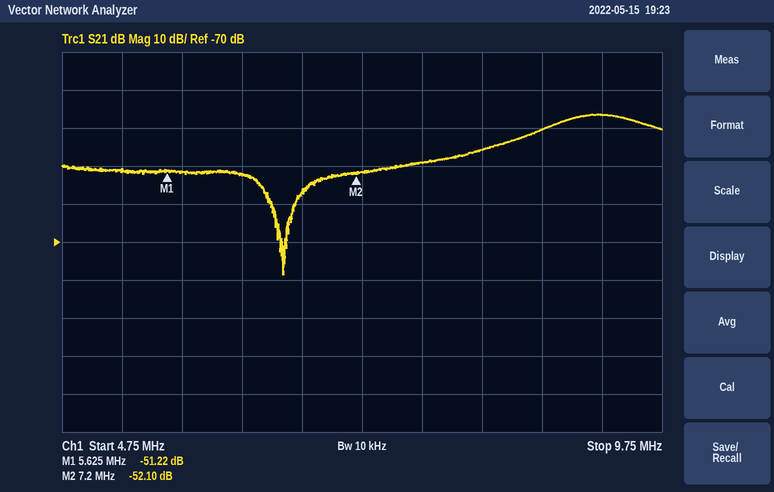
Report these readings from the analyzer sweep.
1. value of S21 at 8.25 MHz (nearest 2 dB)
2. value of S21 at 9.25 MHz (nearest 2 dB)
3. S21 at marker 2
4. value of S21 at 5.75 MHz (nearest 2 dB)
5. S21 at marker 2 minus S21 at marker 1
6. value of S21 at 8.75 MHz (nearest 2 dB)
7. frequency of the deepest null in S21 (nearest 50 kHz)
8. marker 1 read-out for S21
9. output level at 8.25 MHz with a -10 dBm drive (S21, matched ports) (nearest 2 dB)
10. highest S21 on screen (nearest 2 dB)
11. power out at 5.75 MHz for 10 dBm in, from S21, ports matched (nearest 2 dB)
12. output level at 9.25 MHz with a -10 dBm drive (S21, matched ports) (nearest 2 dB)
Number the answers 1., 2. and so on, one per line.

1. -46 dB
2. -36 dB
3. -52.10 dB
4. -52 dB
5. -0.88 dB
6. -40 dB
7. 6.60 MHz
8. -51.22 dB
9. -56 dBm
10. -36 dB
11. -42 dBm
12. -46 dBm
